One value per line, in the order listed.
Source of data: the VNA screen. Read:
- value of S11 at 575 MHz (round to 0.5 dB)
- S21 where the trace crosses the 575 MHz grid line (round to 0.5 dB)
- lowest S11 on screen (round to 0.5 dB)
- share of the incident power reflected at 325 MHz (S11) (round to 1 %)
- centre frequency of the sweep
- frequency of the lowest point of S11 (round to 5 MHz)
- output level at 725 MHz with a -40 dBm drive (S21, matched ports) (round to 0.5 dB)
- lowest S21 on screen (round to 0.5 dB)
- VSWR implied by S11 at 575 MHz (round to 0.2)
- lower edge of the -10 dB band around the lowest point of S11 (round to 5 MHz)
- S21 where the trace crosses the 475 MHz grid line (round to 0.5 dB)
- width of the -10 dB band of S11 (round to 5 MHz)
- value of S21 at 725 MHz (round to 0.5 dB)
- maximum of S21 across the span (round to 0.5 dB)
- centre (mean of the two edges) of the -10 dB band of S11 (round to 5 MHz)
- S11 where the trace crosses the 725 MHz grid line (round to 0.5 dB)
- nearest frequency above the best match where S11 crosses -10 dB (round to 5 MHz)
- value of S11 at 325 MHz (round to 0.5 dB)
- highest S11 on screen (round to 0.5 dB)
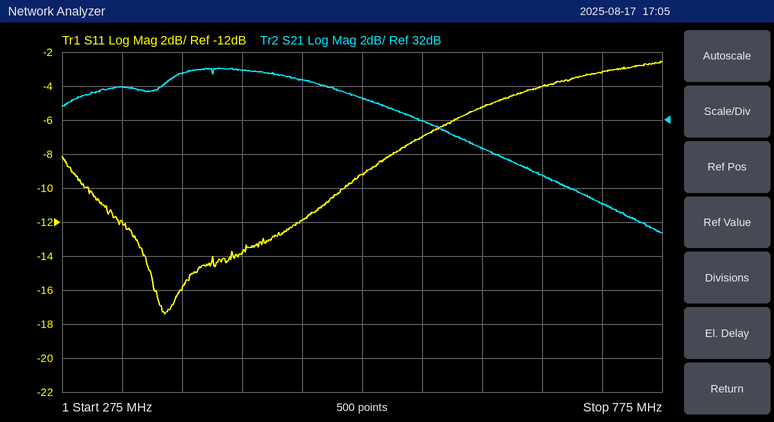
-7.0 dB
32.0 dB
-17.5 dB
6 %
525 MHz
360 MHz
-13.0 dBm
25.5 dB
2.6
295 MHz
34.5 dB
215 MHz
27.0 dB
35.0 dB
405 MHz
-3.0 dB
510 MHz
-12.0 dB
-2.5 dB
